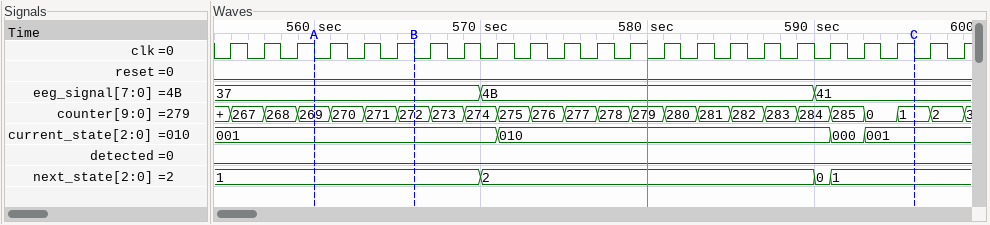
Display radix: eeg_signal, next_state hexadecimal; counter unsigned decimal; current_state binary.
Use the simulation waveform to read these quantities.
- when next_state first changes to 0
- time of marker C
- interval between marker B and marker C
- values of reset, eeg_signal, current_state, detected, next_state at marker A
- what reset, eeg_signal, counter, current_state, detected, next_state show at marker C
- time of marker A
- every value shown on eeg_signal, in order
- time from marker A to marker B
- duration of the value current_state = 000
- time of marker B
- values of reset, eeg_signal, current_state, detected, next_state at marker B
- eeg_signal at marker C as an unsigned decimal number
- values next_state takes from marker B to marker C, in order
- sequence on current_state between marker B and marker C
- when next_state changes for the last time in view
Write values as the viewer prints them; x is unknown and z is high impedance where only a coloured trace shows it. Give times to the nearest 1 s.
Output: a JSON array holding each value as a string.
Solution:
["590 s", "596 s", "30 s", "reset=0, eeg_signal=37, current_state=001, detected=0, next_state=1", "reset=0, eeg_signal=41, counter=1, current_state=001, detected=0, next_state=1", "560 s", "37, 4B, 41", "6 s", "2 s", "566 s", "reset=0, eeg_signal=37, current_state=001, detected=0, next_state=1", "65", "1, 2, 0, 1", "001, 010, 000, 001", "591 s"]
